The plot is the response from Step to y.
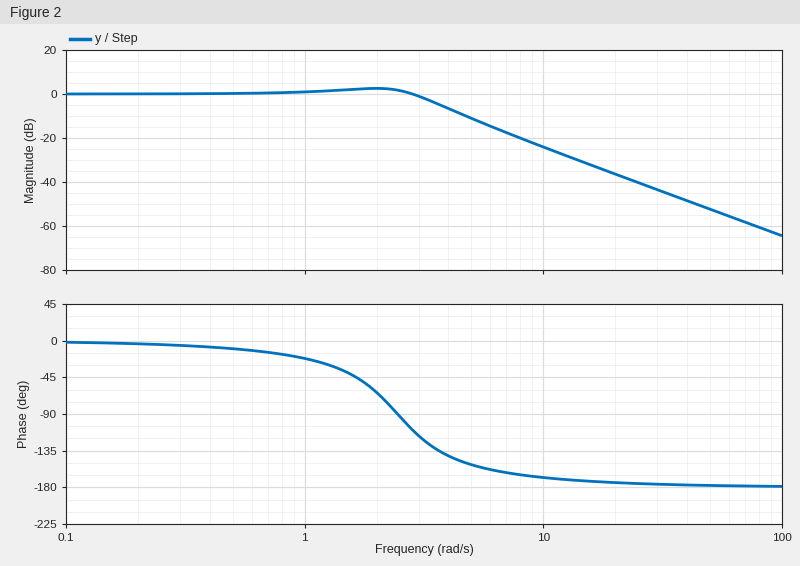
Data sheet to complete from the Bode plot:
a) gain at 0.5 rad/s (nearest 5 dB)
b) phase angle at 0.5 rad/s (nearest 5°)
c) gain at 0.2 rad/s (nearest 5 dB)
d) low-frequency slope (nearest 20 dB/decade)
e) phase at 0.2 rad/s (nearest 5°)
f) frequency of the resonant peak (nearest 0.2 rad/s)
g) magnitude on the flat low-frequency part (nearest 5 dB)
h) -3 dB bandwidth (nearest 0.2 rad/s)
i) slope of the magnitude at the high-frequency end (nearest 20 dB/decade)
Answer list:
0 dB
-10°
0 dB
0 dB/decade
-5°
2.0 rad/s
0 dB
3.4 rad/s
-40 dB/decade
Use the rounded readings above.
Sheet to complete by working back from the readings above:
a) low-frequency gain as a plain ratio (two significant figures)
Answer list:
1.0
